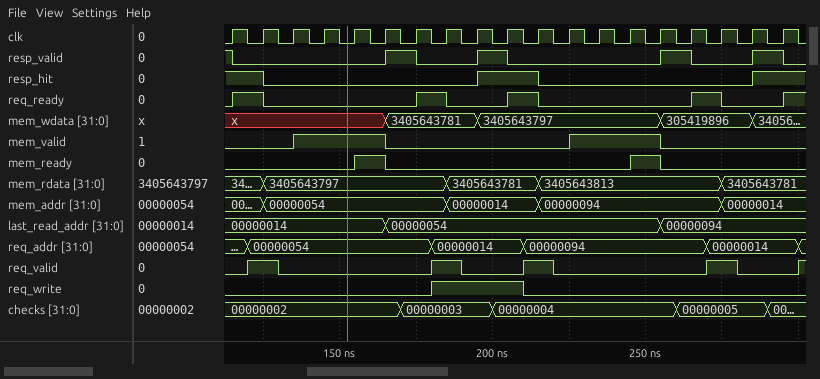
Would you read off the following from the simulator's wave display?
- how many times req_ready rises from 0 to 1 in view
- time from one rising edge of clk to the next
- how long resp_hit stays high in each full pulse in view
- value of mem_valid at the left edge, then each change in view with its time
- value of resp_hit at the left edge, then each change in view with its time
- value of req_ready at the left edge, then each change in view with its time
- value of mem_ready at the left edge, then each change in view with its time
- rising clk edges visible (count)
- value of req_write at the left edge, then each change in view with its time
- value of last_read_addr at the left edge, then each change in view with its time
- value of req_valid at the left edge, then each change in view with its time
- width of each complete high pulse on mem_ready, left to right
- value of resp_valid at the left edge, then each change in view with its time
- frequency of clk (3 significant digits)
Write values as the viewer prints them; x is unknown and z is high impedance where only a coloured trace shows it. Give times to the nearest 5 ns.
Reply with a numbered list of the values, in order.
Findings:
1. 5
2. 10 ns
3. 20 ns
4. 0, 1 at 135 ns, 0 at 165 ns, 1 at 225 ns, 0 at 255 ns
5. 1, 0 at 125 ns, 1 at 195 ns, 0 at 215 ns, 1 at 285 ns
6. 0, 1 at 115 ns, 0 at 125 ns, 1 at 175 ns, 0 at 185 ns, 1 at 205 ns, 0 at 215 ns, 1 at 265 ns, 0 at 275 ns, 1 at 295 ns
7. 0, 1 at 155 ns, 0 at 165 ns, 1 at 245 ns, 0 at 255 ns
8. 19
9. 0, 1 at 180 ns, 0 at 210 ns
10. 00000014, 00000054 at 165 ns, 00000094 at 255 ns
11. 0, 1 at 120 ns, 0 at 130 ns, 1 at 180 ns, 0 at 190 ns, 1 at 210 ns, 0 at 220 ns, 1 at 270 ns, 0 at 280 ns, 1 at 300 ns
12. 10 ns, 10 ns
13. 1, 0 at 115 ns, 1 at 165 ns, 0 at 175 ns, 1 at 195 ns, 0 at 205 ns, 1 at 255 ns, 0 at 265 ns, 1 at 285 ns, 0 at 295 ns
14. 100 MHz
